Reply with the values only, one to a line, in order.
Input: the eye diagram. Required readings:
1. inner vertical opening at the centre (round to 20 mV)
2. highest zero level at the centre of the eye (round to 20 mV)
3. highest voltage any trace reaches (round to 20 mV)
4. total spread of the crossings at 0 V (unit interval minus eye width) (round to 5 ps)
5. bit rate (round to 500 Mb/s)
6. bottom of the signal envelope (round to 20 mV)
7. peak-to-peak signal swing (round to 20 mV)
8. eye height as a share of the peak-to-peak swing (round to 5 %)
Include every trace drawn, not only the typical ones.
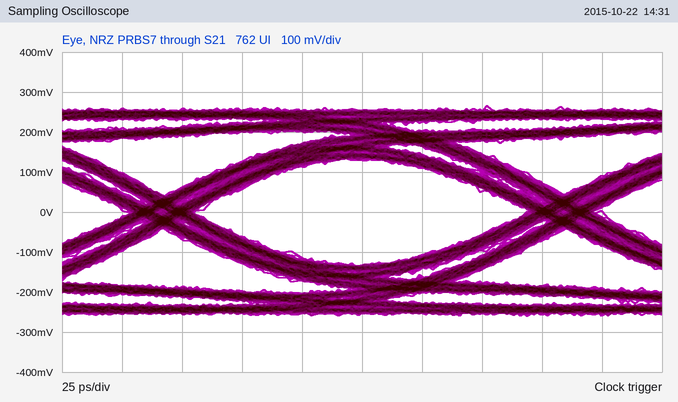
260 mV
-140 mV
260 mV
30 ps
6.0 Gb/s
-260 mV
520 mV
50 %
